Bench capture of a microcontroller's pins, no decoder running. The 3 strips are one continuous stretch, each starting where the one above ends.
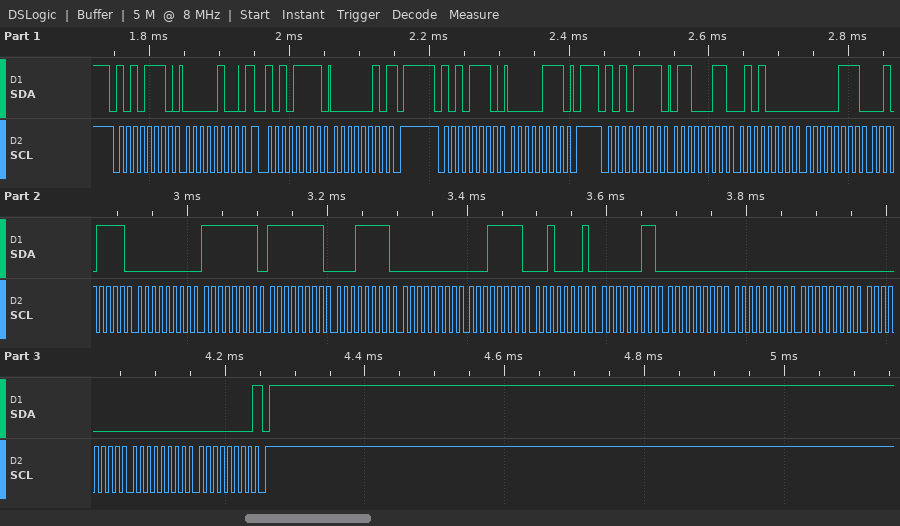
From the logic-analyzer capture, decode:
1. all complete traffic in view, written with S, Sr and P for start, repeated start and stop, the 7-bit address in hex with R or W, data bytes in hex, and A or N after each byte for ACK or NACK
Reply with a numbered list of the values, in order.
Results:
1. S 57W A 04 A Sr 57R A 02 N P S 57W A 07 A P S 57R A 63 A 50 A 07 A 2F A 00 A FF A FF A 1F A 00 A 1F A 21 A 03 A 00 A 00 A 00 A 00 A 00 A 00 N P
